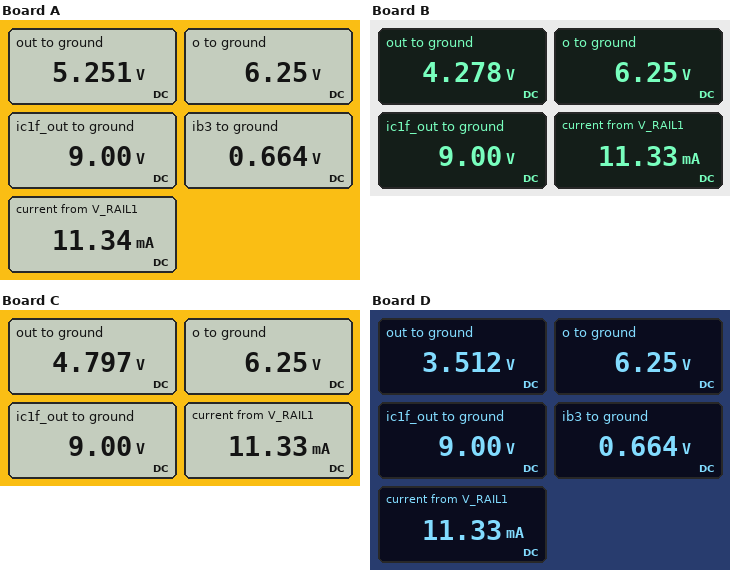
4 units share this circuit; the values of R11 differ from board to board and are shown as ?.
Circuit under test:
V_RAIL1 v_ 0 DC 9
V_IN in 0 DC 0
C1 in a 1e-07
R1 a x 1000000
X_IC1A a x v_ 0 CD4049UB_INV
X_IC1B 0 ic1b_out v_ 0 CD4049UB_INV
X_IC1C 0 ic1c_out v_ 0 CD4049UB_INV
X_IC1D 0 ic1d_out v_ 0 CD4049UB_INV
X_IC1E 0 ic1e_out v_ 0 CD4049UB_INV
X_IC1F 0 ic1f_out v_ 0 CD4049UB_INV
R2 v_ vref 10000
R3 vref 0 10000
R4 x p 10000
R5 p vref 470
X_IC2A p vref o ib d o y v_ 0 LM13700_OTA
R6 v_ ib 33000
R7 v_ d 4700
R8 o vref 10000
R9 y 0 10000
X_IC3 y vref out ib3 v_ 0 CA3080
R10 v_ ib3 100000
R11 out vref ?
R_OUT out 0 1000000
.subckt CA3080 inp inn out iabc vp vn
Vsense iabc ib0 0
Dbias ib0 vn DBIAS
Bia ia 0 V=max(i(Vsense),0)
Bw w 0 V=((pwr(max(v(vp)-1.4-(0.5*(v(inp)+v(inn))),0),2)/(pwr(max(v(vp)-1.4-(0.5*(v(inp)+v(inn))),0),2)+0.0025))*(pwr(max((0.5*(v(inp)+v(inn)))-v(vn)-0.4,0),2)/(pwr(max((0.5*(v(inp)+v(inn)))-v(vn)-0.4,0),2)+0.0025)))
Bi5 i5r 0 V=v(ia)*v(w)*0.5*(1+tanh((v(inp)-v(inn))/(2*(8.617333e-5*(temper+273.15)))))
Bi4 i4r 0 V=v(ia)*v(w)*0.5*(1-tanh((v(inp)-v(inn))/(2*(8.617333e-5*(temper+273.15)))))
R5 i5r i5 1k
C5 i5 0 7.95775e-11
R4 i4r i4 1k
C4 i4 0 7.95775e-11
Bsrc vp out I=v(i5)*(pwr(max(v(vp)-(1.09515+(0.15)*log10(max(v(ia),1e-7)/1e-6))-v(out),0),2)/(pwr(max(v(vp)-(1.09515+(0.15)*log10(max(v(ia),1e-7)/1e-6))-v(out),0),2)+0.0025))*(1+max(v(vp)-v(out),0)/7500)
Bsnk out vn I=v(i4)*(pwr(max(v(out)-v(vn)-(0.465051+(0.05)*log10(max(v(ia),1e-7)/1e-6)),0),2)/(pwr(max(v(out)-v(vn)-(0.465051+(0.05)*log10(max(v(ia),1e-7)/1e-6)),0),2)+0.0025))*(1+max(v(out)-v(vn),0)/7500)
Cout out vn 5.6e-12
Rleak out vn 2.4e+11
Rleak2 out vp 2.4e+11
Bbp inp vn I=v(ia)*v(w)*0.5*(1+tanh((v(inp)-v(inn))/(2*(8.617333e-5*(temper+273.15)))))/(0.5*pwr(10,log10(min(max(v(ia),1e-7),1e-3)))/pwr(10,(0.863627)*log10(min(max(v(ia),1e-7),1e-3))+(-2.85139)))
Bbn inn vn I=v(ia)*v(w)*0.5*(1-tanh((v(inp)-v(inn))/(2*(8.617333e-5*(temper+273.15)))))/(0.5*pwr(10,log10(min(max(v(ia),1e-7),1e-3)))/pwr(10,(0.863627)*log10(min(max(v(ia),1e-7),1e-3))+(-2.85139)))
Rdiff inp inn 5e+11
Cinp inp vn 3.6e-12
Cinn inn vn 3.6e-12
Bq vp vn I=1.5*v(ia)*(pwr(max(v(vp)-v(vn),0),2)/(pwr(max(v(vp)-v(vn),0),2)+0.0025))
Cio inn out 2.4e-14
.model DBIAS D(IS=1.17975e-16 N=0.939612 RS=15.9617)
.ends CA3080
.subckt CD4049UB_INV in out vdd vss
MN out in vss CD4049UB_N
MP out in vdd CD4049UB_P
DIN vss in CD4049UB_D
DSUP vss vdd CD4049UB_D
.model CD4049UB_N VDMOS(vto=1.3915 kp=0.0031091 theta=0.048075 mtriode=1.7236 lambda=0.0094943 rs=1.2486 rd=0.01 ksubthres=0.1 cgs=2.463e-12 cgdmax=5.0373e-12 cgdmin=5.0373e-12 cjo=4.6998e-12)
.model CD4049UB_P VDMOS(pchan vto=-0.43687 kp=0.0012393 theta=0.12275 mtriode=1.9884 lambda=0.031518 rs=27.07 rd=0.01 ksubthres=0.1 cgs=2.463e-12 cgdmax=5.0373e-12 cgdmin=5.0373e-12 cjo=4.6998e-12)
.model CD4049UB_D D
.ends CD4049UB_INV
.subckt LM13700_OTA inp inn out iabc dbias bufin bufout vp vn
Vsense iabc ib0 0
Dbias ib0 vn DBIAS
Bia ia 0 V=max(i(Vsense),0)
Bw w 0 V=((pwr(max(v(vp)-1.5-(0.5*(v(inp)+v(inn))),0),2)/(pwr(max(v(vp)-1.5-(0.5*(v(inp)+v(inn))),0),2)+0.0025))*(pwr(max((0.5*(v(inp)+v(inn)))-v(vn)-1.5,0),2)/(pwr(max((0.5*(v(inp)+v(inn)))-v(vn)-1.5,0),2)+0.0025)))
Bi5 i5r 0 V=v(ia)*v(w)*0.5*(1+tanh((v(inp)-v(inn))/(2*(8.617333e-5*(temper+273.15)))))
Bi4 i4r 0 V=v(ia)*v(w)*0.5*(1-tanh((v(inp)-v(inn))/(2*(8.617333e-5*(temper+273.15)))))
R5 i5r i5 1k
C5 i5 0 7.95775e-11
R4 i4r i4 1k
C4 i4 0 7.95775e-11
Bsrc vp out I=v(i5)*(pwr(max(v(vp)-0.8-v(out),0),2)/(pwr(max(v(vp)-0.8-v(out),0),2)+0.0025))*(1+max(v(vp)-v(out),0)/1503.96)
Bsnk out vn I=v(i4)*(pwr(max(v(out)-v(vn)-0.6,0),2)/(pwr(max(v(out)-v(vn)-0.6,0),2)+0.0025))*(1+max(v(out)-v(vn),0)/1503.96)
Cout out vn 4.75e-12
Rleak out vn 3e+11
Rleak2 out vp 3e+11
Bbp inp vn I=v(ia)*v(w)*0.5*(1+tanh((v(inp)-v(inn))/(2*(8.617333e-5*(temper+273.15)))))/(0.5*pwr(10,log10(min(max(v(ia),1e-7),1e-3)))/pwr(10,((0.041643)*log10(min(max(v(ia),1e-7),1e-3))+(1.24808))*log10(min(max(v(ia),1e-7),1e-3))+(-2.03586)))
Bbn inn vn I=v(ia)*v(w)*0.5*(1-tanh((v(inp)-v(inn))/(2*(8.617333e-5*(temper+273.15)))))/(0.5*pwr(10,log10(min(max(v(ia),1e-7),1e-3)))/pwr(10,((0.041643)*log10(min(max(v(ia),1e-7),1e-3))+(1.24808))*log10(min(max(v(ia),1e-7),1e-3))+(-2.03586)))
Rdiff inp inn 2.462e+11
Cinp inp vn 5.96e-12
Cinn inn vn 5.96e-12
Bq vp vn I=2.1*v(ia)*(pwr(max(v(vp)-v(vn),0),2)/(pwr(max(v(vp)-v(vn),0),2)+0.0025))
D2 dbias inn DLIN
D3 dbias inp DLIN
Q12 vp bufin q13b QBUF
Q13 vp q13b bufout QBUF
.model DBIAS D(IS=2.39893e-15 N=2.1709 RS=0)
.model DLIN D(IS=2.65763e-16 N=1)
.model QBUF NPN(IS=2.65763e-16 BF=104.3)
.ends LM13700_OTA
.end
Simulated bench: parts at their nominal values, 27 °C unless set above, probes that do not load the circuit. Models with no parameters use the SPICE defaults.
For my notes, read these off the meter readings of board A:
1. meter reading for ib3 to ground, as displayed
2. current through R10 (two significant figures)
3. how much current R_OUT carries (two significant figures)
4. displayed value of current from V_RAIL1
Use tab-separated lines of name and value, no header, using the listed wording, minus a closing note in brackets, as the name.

meter reading for ib3 to ground, as displayed	0.664 V
current through R10	83 µA
how much current R_OUT carries	5.3 µA
displayed value of current from V_RAIL1	11.34 mA
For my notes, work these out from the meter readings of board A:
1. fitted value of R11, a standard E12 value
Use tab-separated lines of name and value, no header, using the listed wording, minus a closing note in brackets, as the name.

fitted value of R11, a standard E12 value	6.8 kΩ
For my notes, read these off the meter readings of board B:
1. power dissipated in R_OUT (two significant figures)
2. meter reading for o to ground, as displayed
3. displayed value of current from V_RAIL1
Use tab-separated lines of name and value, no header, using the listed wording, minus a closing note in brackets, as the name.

power dissipated in R_OUT	18 µW
meter reading for o to ground, as displayed	6.25 V
displayed value of current from V_RAIL1	11.33 mA
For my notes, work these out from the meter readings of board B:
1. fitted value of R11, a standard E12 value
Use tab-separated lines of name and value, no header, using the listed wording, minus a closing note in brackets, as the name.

fitted value of R11, a standard E12 value	18 kΩ
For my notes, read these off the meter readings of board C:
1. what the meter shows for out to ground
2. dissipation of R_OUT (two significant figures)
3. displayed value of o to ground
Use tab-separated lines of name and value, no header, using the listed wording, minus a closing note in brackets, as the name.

what the meter shows for out to ground	4.797 V
dissipation of R_OUT	23 µW
displayed value of o to ground	6.25 V
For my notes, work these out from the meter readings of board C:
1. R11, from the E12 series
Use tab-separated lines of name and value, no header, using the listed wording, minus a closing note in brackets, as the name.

R11, from the E12 series	12 kΩ
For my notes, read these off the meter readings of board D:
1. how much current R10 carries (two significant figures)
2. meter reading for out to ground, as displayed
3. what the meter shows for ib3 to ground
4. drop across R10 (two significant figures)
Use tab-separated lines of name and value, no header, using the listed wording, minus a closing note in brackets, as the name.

how much current R10 carries	83 µA
meter reading for out to ground, as displayed	3.512 V
what the meter shows for ib3 to ground	0.664 V
drop across R10	8.3 V
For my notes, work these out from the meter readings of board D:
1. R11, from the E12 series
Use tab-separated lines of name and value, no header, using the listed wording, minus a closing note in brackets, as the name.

R11, from the E12 series	27 kΩ
